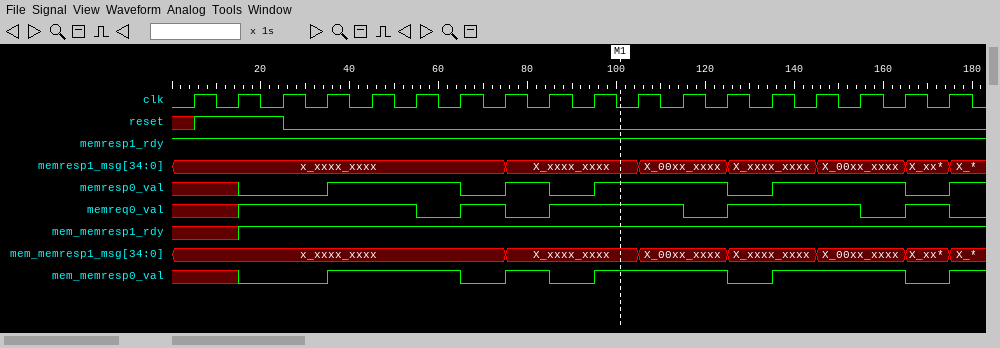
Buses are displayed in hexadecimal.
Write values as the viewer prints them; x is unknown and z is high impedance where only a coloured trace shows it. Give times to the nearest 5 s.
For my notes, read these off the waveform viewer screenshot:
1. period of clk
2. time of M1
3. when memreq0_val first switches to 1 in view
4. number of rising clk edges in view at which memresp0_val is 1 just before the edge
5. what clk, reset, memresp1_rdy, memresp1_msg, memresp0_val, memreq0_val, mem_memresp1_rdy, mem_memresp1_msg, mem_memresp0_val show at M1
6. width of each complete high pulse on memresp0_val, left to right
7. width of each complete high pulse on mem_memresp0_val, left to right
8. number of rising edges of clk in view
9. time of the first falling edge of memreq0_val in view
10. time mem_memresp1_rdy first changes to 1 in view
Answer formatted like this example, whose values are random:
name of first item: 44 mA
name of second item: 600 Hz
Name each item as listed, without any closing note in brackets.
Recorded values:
period of clk: 10 s
time of M1: 100 s
when memreq0_val first switches to 1 in view: 15 s
number of rising clk edges in view at which memresp0_val is 1 just before the edge: 10
what clk, reset, memresp1_rdy, memresp1_msg, memresp0_val, memreq0_val, mem_memresp1_rdy, mem_memresp1_msg, mem_memresp0_val show at M1: clk=0, reset=0, memresp1_rdy=1, memresp1_msg=X_xxxx_xxxx, memresp0_val=1, memreq0_val=1, mem_memresp1_rdy=1, mem_memresp1_msg=X_xxxx_xxxx, mem_memresp0_val=1
width of each complete high pulse on memresp0_val, left to right: 30 s, 10 s, 30 s, 30 s
width of each complete high pulse on mem_memresp0_val, left to right: 30 s, 10 s, 30 s, 30 s
number of rising edges of clk in view: 18
time of the first falling edge of memreq0_val in view: 55 s
time mem_memresp1_rdy first changes to 1 in view: 15 s
